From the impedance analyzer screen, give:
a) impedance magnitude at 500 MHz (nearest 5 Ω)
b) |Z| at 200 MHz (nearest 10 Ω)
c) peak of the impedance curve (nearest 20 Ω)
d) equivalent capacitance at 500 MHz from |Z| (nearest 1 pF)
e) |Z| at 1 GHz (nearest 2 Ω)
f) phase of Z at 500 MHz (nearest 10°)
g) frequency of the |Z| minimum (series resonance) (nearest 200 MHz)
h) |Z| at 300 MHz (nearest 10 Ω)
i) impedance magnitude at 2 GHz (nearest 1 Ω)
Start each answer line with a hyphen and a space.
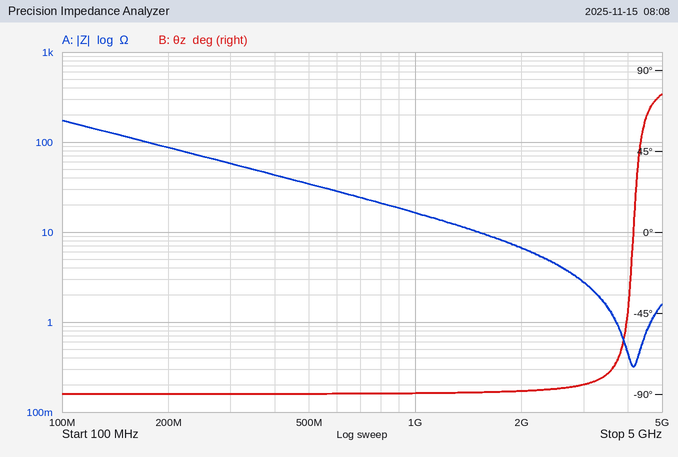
- 35 Ω
- 90 Ω
- 180 Ω
- 9 pF
- 16 Ω
- -90°
- 4.2 GHz
- 60 Ω
- 7 Ω
